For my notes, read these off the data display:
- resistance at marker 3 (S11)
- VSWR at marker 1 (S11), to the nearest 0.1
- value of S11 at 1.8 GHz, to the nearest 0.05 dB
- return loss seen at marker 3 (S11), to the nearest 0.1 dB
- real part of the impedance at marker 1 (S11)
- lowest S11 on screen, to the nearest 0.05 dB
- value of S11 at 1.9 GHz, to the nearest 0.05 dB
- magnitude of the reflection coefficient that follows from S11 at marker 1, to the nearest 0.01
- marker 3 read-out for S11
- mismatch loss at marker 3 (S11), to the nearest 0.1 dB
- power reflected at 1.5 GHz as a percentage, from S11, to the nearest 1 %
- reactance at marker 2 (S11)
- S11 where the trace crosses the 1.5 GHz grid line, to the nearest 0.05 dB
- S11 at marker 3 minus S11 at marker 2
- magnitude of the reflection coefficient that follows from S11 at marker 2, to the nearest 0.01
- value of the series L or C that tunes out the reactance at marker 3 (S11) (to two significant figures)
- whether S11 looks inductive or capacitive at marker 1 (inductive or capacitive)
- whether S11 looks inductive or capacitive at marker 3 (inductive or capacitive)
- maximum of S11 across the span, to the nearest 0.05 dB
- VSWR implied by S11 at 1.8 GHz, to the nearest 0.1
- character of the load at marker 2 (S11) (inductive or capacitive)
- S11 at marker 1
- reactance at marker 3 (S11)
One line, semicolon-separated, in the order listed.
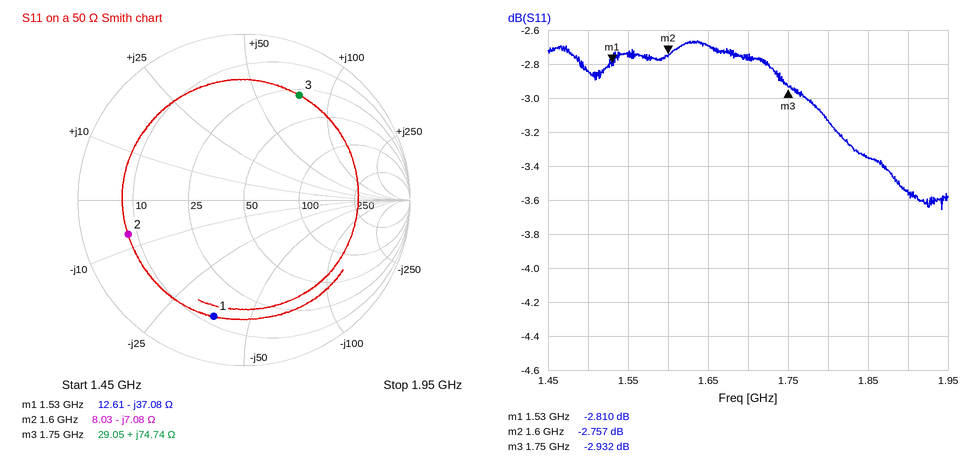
29.05 Ω; 6.2; -3.15 dB; 2.9 dB; 12.61 Ω; -3.65 dB; -3.55 dB; 0.72; -2.932 dB; 3.1 dB; 52 %; -7.08 Ω; -2.85 dB; -0.175 dB; 0.73; 1.2 pF; capacitive; inductive; -2.65 dB; 5.6; capacitive; -2.810 dB; +74.74 Ω
